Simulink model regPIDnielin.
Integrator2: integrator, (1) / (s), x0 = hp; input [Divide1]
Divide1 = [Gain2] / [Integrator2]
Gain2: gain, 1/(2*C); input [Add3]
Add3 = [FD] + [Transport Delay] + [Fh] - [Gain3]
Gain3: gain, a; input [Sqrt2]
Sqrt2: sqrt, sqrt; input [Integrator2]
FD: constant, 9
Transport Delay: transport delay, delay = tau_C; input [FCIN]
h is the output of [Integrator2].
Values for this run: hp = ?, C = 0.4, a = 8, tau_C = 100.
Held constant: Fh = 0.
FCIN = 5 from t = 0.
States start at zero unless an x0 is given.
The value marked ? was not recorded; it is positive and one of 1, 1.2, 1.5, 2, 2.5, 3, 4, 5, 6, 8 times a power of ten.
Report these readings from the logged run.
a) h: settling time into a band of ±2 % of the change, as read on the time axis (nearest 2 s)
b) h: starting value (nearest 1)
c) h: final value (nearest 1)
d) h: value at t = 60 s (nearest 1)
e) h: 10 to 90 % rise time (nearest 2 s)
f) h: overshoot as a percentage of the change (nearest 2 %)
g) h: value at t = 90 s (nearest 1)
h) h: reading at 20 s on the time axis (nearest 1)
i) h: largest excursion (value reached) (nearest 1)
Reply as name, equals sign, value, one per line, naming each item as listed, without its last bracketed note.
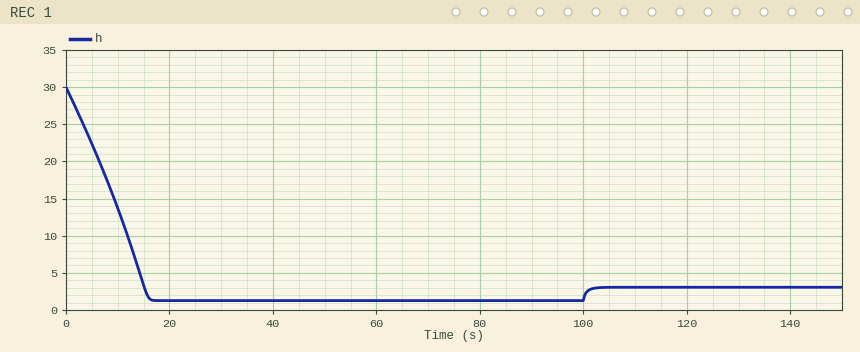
h: settling time into a band of ±2 % of the change, as read on the time axis = 100 s
h: starting value = 30
h: final value = 3
h: value at t = 60 s = 1
h: 10 to 90 % rise time = 12 s
h: overshoot as a percentage of the change = 6 %
h: value at t = 90 s = 1
h: reading at 20 s on the time axis = 1
h: largest excursion (value reached) = 1
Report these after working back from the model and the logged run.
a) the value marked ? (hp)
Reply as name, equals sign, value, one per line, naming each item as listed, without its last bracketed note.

the value marked ? = 30
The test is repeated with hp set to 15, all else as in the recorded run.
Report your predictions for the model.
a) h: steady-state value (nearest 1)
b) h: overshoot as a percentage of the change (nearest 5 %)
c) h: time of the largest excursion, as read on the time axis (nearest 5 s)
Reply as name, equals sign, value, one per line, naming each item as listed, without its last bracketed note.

h: steady-state value = 3
h: overshoot as a percentage of the change = 15 %
h: time of the largest excursion, as read on the time axis = 15 s
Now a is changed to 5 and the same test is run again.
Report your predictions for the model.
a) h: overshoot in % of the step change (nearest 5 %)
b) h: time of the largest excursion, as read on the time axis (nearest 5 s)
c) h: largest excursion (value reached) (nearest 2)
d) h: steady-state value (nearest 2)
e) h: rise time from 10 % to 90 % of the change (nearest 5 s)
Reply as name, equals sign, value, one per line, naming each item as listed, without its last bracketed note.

h: overshoot in % of the step change = 20 %
h: time of the largest excursion, as read on the time axis = 95 s
h: largest excursion (value reached) = 4
h: steady-state value = 8
h: rise time from 10 % to 90 % of the change = 20 s
